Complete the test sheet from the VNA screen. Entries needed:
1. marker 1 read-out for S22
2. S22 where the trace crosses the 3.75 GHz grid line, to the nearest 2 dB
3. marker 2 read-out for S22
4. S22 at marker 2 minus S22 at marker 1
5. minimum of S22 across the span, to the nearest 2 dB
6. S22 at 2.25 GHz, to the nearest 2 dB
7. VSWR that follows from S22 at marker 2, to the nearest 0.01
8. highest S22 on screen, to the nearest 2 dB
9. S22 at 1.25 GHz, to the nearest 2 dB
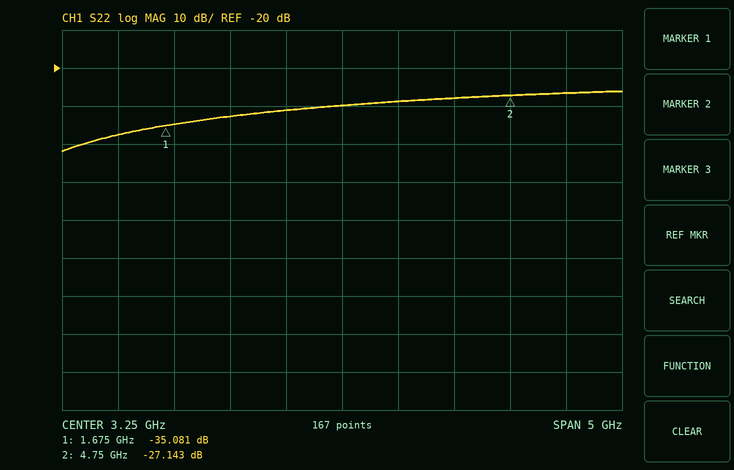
-35.081 dB
-28 dB
-27.143 dB
7.938 dB
-42 dB
-32 dB
1.09
-26 dB
-38 dB
